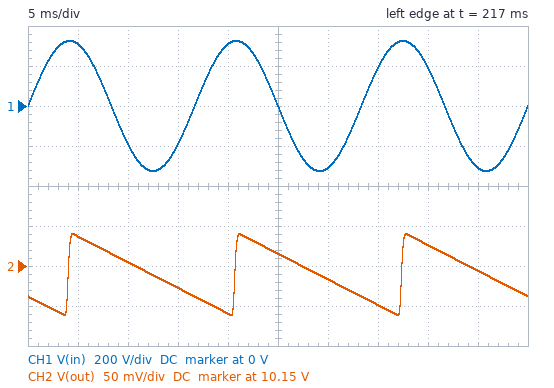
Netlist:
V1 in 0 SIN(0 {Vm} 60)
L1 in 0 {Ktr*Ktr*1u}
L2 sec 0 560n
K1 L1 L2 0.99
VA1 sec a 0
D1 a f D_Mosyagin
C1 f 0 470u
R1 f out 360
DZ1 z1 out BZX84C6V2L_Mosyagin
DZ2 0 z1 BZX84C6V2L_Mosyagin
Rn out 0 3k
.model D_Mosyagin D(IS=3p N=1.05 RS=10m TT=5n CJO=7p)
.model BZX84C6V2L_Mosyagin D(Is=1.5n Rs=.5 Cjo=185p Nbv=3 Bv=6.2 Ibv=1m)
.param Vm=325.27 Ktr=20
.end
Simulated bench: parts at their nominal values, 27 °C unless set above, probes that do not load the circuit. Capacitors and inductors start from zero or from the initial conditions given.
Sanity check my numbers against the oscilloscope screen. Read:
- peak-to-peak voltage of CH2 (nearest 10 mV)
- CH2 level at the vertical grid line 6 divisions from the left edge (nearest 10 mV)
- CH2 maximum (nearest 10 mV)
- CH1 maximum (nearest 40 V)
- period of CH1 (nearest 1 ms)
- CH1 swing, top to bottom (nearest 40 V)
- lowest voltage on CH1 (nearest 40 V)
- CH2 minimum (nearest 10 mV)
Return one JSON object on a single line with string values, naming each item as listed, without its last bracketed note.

{"peak-to-peak voltage of CH2": "100 mV", "CH2 level at the vertical grid line 6 divisions from the left edge": "10.13 V", "CH2 maximum": "10.19 V", "CH1 maximum": "320 V", "period of CH1": "17 ms", "CH1 swing, top to bottom": "640 V", "lowest voltage on CH1": "-320 V", "CH2 minimum": "10.09 V"}
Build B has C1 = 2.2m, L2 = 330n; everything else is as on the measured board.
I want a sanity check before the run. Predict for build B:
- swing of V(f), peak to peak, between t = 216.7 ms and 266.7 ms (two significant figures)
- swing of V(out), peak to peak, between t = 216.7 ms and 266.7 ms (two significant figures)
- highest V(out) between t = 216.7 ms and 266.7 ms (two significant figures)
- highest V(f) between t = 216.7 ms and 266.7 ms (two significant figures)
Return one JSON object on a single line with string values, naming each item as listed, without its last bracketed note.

{"swing of V(f), peak to peak, between t = 216.7 ms and 266.7 ms": "18 mV", "swing of V(out), peak to peak, between t = 216.7 ms and 266.7 ms": "16 mV", "highest V(out) between t = 216.7 ms and 266.7 ms": "7.7 V", "highest V(f) between t = 216.7 ms and 266.7 ms": "8.6 V"}
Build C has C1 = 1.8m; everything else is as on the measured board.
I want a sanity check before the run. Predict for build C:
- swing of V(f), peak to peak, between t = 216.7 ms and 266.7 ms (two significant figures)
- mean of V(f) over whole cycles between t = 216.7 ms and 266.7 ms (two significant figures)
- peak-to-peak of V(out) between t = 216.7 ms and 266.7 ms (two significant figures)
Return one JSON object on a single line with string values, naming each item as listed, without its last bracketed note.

{"swing of V(f), peak to peak, between t = 216.7 ms and 266.7 ms": "30 mV", "mean of V(f) over whole cycles between t = 216.7 ms and 266.7 ms": "11 V", "peak-to-peak of V(out) between t = 216.7 ms and 266.7 ms": "27 mV"}
